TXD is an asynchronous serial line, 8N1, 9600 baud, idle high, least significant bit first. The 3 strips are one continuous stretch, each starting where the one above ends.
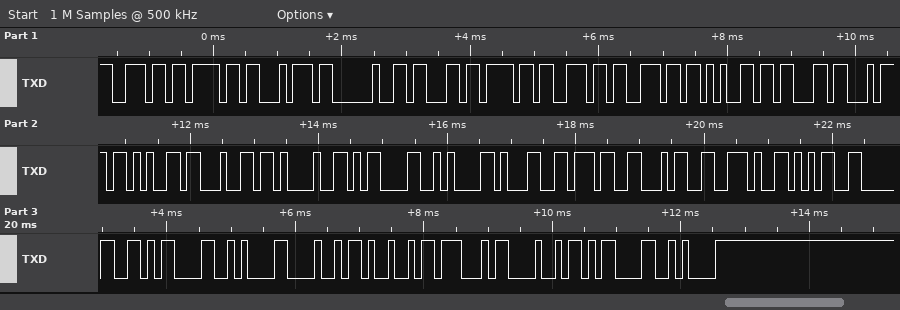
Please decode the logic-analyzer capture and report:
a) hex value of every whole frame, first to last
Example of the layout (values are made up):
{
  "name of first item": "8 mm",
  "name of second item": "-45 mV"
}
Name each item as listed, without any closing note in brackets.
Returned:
{
  "hex value of every whole frame, first to last": "6E 6F 74 20 63 6F 6E 6E 65 63 74 65 64 21 0D 0A 31 37 34 2E 35 30 0D 0A 48 49 47 48 0D 0A"
}
